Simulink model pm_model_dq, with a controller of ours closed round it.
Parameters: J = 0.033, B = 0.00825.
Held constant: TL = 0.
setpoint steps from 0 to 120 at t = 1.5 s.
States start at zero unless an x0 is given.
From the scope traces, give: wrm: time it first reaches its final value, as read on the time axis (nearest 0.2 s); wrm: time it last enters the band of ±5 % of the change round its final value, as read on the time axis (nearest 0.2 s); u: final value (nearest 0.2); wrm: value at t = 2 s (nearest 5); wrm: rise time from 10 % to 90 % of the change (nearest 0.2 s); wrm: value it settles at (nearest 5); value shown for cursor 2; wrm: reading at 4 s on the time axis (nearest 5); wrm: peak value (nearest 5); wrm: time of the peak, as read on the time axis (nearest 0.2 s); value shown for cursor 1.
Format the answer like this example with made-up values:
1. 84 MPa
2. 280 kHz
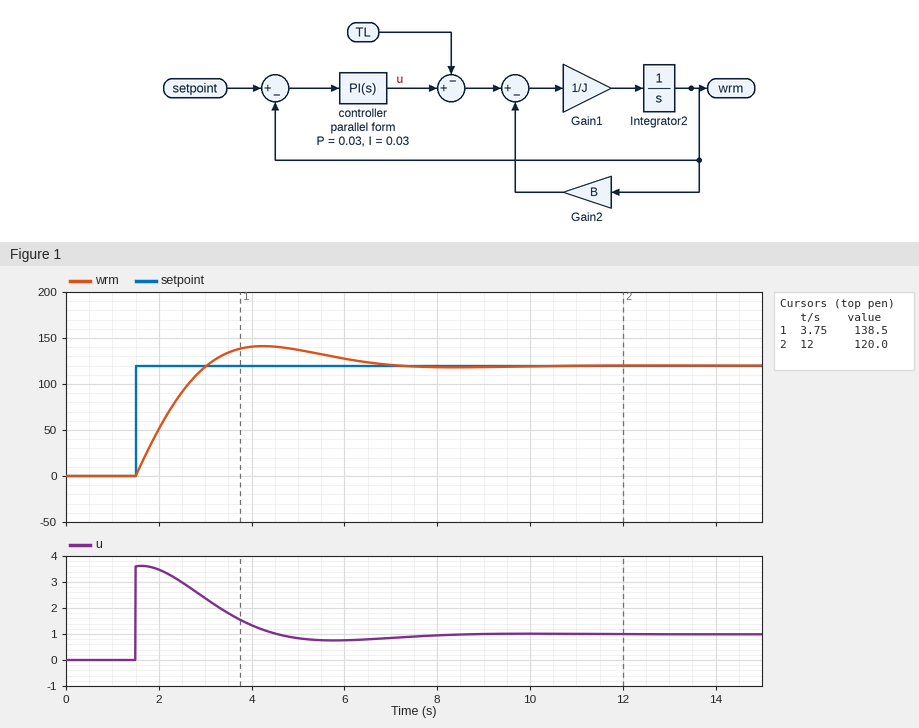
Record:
1. 3.0 s
2. 6.2 s
3. 1.0
4. 50
5. 1.2 s
6. 120
7. 120.0
8. 140
9. 140
10. 4.2 s
11. 138.5
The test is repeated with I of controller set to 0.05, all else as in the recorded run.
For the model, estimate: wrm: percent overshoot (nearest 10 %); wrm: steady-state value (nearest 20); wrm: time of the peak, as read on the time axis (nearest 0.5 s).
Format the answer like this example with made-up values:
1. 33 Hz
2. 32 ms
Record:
1. 30 %
2. 120
3. 3.5 s
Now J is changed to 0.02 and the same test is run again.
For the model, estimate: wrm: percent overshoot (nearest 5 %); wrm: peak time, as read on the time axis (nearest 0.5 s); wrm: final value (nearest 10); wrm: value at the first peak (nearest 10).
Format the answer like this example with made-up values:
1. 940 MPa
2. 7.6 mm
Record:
1. 10 %
2. 3.5 s
3. 120
4. 130
